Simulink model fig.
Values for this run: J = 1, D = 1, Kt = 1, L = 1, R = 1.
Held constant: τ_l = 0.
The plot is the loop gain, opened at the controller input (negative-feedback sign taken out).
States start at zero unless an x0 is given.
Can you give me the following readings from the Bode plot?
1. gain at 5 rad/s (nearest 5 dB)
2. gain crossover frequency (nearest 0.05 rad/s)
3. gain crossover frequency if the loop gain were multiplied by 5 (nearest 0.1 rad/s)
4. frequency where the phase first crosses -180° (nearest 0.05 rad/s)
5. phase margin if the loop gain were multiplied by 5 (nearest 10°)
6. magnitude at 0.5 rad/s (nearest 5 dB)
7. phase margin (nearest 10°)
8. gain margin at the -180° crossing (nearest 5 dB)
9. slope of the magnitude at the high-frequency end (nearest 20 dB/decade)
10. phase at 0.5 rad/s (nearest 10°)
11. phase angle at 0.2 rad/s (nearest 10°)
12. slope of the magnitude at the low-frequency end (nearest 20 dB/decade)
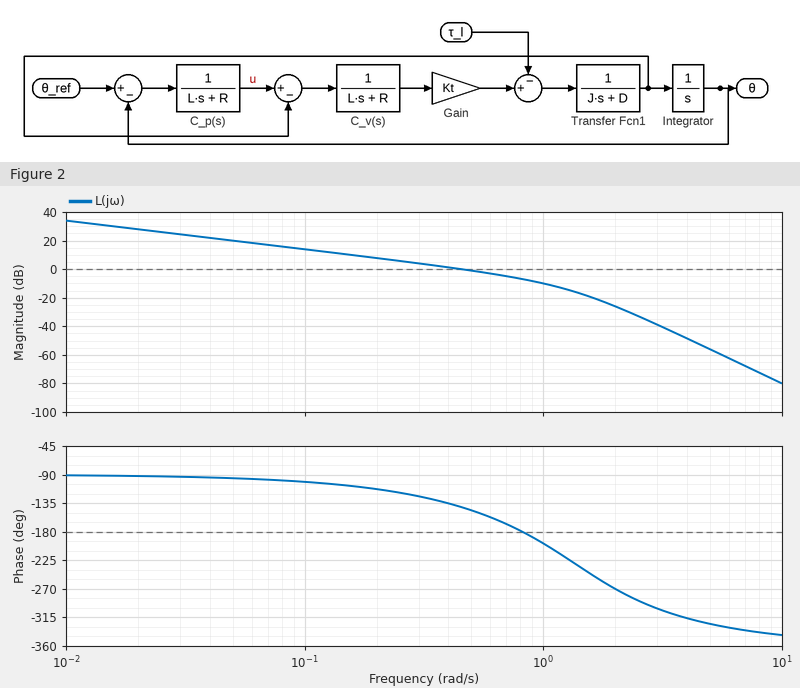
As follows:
-55 dB
0.45 rad/s
1.2 rad/s
0.80 rad/s
-40°
0 dB
40°
5 dB
-80 dB/decade
-150°
-110°
-20 dB/decade
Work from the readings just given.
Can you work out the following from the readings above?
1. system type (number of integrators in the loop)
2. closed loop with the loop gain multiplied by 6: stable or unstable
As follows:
1
unstable
